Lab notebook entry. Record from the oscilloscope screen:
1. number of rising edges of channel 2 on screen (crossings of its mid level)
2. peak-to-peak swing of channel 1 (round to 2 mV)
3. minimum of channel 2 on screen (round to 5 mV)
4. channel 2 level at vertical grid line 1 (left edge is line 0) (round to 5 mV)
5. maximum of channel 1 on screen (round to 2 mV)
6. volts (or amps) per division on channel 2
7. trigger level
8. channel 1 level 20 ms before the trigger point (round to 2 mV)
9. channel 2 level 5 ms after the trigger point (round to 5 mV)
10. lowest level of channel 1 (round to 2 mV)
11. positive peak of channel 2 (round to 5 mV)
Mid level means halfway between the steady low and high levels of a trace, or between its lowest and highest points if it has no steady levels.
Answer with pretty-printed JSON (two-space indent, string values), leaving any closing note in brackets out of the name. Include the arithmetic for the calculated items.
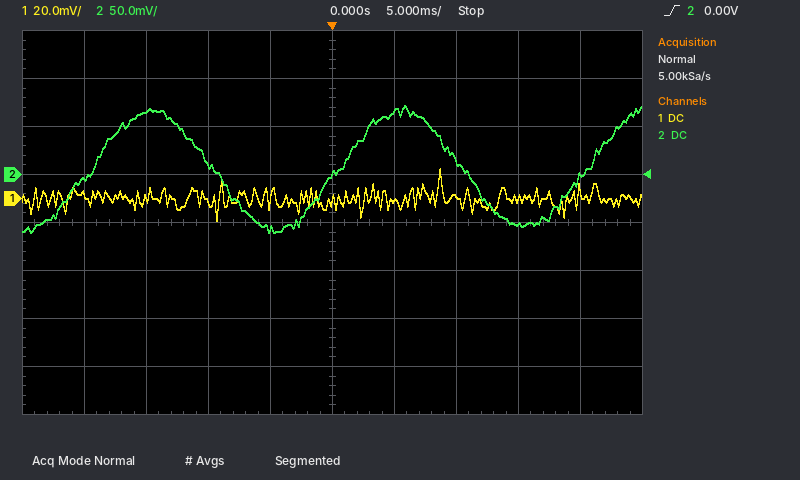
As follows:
{
  "number of rising edges of channel 2 on screen": "3",
  "peak-to-peak swing of channel 1": "12 mV − (-10 mV) = 22 mV",
  "minimum of channel 2 on screen": "-60 mV",
  "channel 2 level at vertical grid line 1 (left edge is line 0)": "-5 mV",
  "maximum of channel 1 on screen": "12 mV",
  "volts (or amps) per division on channel 2": "50 mV",
  "trigger level": "0.00 V",
  "channel 1 level 20 ms before the trigger point": "2 mV",
  "channel 2 level 5 ms after the trigger point": "65 mV",
  "lowest level of channel 1": "-10 mV",
  "positive peak of channel 2": "70 mV"
}
